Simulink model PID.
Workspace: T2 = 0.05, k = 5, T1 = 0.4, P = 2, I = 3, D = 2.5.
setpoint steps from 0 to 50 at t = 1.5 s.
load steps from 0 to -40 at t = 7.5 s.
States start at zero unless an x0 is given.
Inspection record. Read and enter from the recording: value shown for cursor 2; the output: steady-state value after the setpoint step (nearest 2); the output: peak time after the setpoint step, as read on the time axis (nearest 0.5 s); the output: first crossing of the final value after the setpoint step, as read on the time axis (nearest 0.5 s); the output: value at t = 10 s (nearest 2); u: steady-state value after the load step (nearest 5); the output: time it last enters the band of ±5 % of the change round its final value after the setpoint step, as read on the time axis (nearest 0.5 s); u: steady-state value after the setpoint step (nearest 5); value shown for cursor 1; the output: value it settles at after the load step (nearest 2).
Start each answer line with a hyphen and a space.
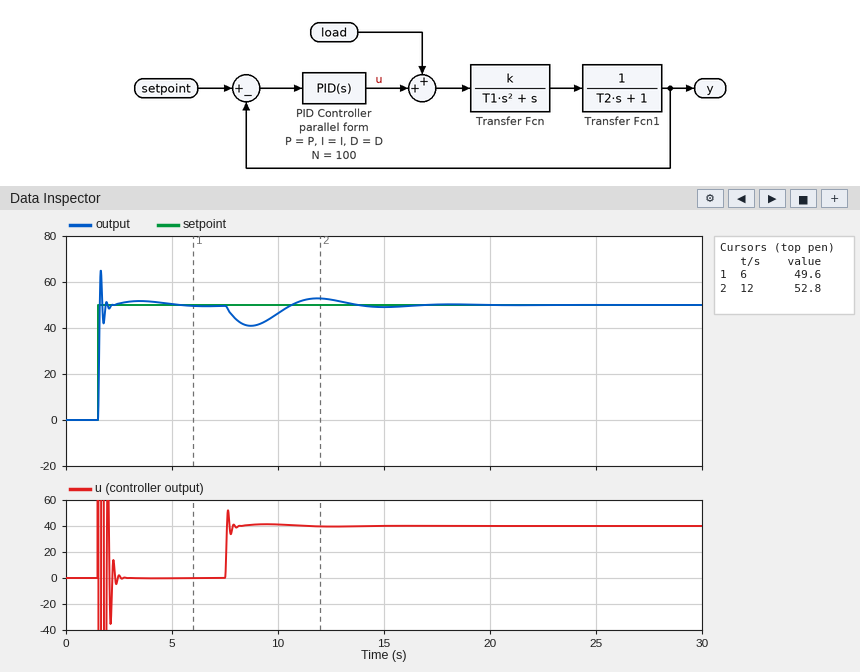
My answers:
- 52.8
- 50
- 1.5 s
- 1.5 s
- 46
- 40
- 2.0 s
- 0
- 49.6
- 50
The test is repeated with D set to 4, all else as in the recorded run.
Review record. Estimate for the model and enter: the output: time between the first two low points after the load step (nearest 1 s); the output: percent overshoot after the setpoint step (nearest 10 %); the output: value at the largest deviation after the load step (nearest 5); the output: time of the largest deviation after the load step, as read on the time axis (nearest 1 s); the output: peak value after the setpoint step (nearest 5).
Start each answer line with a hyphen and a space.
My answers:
- 8 s
- 50 %
- 40
- 9 s
- 75
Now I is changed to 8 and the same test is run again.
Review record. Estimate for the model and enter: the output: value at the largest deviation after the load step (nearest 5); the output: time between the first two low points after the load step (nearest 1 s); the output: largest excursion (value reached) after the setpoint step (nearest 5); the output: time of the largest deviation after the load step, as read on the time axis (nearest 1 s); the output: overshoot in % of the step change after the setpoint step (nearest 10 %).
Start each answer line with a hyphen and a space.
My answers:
- 45
- 4 s
- 65
- 8 s
- 30 %
